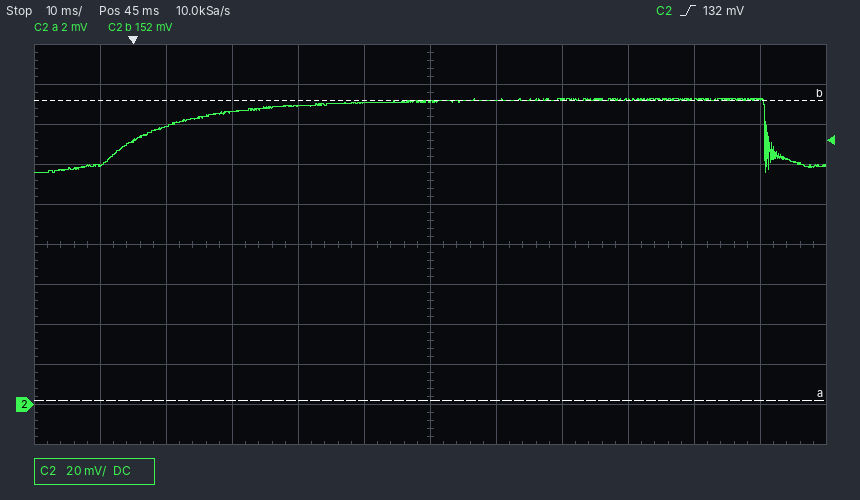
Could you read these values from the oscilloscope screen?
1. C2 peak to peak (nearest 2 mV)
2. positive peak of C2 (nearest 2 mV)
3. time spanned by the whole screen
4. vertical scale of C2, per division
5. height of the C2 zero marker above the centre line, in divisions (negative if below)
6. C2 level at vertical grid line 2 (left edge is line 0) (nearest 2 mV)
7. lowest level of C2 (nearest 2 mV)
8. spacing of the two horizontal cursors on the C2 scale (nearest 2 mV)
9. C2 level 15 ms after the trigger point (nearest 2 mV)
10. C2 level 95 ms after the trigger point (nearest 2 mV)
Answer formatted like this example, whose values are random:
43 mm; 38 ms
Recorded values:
36 mV; 152 mV; 120 ms; 20 mV; -4.0 div; 140 mV; 116 mV; 150 mV; 146 mV; 152 mV
